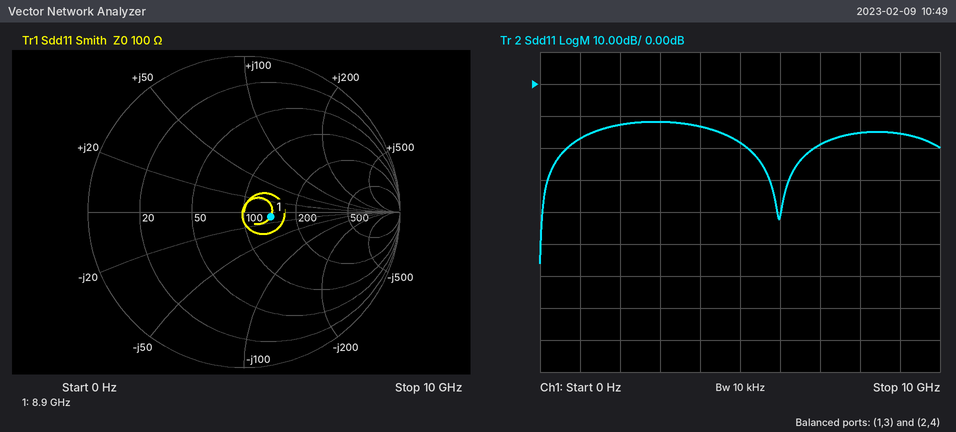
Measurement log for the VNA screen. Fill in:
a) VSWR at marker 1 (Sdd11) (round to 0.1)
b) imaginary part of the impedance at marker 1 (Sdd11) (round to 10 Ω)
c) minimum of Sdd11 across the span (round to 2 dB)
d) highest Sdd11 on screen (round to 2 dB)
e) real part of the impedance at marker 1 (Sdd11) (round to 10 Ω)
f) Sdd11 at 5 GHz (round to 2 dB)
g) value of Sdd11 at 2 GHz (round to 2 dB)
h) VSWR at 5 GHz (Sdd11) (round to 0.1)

1.4
-10 Ω
-56 dB
-12 dB
140 Ω
-18 dB
-12 dB
1.3
